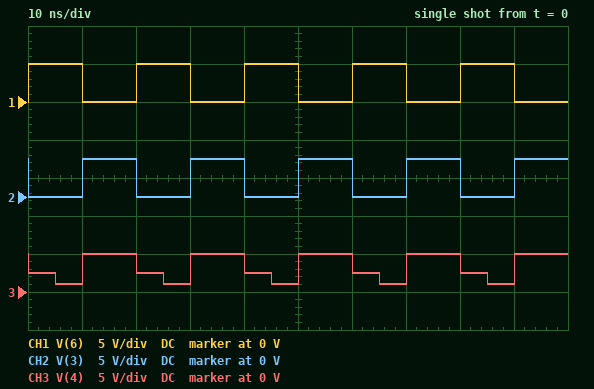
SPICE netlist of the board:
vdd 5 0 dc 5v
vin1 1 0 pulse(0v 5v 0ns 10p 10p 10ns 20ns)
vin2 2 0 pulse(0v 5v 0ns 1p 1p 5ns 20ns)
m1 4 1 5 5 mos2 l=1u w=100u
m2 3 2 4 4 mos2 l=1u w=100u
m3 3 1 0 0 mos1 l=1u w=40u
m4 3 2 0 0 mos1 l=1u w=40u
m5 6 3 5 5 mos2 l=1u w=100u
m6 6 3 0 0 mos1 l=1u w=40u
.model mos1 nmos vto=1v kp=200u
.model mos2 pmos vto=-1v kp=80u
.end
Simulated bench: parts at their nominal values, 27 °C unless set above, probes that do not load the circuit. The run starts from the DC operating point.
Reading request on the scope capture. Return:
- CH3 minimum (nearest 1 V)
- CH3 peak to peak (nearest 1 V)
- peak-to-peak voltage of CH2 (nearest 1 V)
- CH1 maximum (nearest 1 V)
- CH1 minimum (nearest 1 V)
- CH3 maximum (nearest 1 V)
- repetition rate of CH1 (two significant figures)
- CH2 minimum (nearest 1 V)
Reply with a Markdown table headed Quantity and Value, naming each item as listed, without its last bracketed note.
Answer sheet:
| Quantity | Value |
|---|---|
| CH3 minimum | 1 V |
| CH3 peak to peak | 4 V |
| peak-to-peak voltage of CH2 | 5 V |
| CH1 maximum | 5 V |
| CH1 minimum | 0 V |
| CH3 maximum | 5 V |
| repetition rate of CH1 | 50 MHz |
| CH2 minimum | 0 V |
